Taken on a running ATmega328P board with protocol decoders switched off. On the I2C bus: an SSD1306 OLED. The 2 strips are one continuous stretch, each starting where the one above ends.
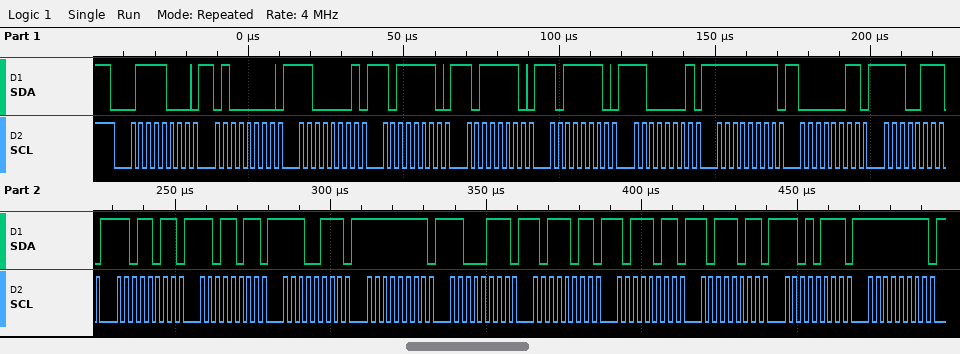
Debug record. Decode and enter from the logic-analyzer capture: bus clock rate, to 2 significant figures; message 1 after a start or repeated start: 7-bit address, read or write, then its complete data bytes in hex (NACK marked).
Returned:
400 kHz
0x3C write: 40 C1 BE BE BE C1 FF 03 E7 DB DB E7 FF C7 BB BB BB D7 FF
